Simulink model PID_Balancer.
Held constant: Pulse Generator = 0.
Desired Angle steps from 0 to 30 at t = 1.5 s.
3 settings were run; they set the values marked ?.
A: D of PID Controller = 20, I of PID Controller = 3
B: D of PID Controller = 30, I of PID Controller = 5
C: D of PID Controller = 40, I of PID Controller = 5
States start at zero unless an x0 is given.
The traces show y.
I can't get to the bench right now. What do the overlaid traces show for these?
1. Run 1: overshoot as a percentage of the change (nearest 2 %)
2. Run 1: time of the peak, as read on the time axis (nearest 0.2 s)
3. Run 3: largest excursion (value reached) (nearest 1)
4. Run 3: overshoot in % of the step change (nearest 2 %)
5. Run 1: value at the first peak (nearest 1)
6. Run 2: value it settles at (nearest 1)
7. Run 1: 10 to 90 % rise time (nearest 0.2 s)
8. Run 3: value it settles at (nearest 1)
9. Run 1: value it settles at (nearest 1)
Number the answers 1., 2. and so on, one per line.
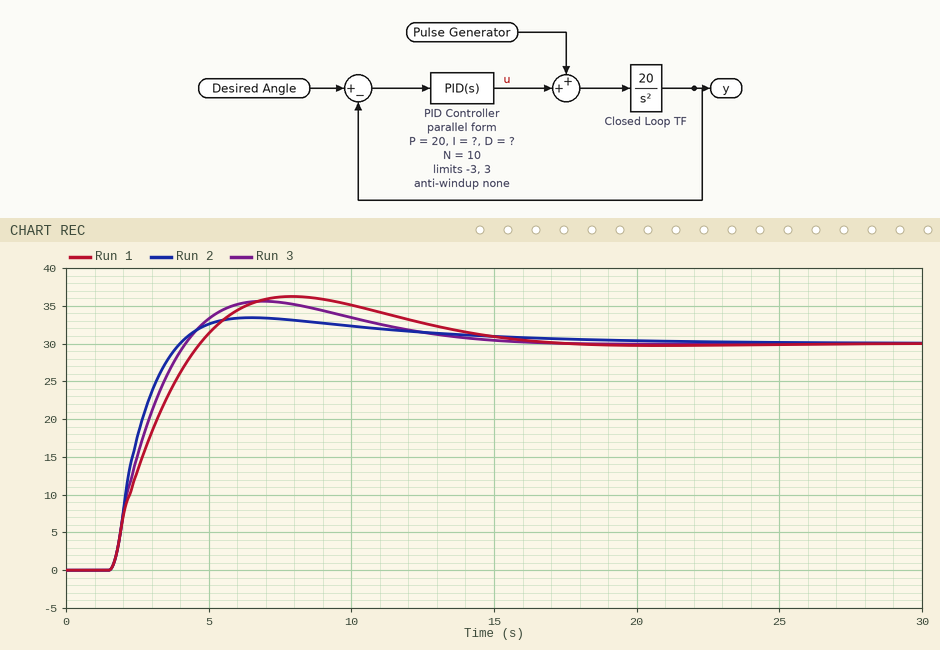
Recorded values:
1. 20 %
2. 8.0 s
3. 36
4. 18 %
5. 36
6. 30
7. 2.4 s
8. 30
9. 30
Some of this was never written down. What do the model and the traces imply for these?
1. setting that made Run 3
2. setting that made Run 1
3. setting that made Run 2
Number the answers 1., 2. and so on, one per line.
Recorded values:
1. B
2. C
3. A
